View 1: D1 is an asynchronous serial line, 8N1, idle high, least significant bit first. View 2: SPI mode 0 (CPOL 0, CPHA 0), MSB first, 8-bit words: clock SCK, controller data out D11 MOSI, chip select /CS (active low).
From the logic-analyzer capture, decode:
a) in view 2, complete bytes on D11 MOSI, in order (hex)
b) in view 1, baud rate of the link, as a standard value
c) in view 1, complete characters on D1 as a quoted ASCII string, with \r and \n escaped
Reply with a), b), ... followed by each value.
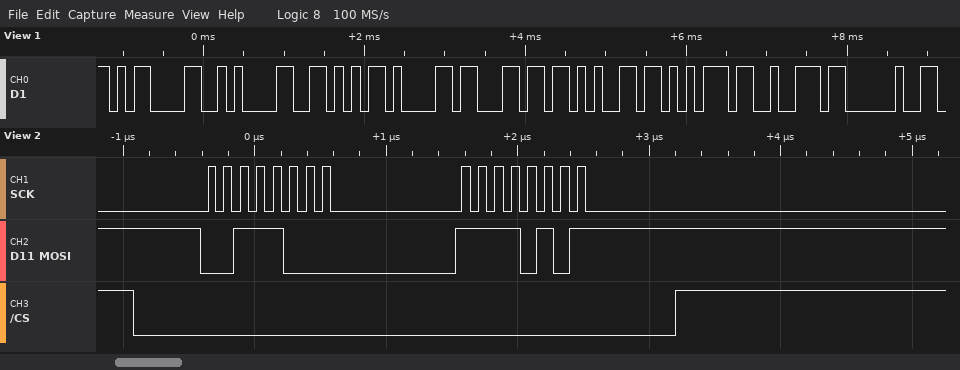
a) 38 F5
b) 9600 baud
c) "\r\nValeur "
